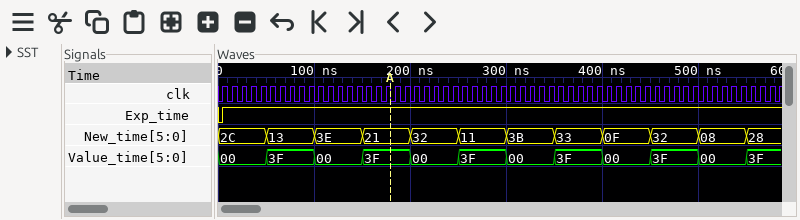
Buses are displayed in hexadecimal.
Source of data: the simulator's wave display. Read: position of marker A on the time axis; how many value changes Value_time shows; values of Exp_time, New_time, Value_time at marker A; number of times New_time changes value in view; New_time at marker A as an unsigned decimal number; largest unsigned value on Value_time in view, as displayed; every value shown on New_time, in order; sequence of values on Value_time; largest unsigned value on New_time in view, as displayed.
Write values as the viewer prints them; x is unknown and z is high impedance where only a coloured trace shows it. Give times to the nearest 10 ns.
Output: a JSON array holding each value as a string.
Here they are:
["180 ns", "11", "Exp_time=1, New_time=21, Value_time=3F", "11", "33", "3F", "2C, 13, 3E, 21, 32, 11, 3B, 33, 0F, 32, 08, 28", "00, 3F, 00, 3F, 00, 3F, 00, 3F, 00, 3F, 00, 3F", "3E"]
